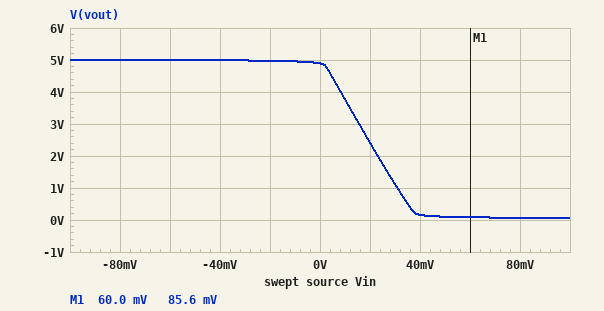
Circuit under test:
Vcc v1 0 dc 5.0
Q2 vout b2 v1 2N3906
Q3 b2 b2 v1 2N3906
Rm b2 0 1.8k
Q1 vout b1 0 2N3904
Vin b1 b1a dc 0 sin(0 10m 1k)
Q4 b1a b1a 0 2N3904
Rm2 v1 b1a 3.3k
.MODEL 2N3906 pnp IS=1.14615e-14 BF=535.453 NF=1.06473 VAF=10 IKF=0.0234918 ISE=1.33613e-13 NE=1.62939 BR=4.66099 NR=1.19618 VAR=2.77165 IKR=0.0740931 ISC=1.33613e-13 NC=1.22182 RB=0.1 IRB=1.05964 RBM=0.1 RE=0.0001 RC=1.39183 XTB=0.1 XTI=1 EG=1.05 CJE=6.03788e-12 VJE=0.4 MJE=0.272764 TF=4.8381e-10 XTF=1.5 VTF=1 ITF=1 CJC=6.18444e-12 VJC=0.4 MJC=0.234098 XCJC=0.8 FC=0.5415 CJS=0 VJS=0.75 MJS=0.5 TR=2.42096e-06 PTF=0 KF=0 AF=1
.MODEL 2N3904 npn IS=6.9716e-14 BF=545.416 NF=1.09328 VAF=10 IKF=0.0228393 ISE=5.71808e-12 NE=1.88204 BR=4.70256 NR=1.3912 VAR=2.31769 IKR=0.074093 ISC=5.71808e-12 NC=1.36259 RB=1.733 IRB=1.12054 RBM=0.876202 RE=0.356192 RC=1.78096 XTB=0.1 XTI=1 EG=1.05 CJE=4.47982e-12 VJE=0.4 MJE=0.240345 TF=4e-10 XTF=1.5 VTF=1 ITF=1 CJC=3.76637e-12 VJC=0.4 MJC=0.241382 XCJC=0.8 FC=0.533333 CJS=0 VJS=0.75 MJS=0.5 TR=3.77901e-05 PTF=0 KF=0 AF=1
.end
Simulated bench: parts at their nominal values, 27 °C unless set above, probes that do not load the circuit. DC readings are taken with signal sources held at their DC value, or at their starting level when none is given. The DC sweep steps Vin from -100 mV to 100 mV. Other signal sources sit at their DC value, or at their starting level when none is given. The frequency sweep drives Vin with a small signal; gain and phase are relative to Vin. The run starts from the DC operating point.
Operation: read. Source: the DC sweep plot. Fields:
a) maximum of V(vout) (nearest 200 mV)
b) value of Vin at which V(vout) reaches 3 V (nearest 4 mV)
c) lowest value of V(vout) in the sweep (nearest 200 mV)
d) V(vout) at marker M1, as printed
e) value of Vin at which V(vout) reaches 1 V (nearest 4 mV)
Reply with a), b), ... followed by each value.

a) 5.0 V
b) 16 mV
c) 0 V
d) 85.6 mV
e) 32 mV
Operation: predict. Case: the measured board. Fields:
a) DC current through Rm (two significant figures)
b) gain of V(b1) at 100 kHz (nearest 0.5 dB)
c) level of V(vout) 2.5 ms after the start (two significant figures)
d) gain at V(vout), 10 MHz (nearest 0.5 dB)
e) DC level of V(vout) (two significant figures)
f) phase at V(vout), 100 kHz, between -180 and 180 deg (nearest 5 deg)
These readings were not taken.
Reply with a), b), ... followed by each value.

a) 2.4 mA
b) 0 dB
c) 4.9 V
d) 1.0 dB
e) 4.9 V
f) 170 deg
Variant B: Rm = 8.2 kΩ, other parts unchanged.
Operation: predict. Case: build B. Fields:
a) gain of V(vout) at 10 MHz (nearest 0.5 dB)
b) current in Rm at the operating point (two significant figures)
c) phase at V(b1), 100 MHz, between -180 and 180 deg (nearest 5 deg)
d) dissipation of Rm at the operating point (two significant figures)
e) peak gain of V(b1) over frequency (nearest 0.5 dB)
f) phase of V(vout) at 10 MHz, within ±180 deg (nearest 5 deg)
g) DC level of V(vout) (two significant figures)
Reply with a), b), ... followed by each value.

a) -5.5 dB
b) 530 µA
c) 0 deg
d) 2.3 mW
e) -5.0 dB
f) 15 deg
g) 68 mV
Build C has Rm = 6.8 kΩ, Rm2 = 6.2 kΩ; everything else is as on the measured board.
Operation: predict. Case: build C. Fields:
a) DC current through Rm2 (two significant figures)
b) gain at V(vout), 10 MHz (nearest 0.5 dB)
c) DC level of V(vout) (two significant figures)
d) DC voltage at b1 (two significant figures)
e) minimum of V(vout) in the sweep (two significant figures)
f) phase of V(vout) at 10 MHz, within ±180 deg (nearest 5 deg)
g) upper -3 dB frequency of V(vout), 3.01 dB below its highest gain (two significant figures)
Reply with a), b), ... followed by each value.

a) 700 µA
b) 29.0 dB
c) 2.0 V
d) 660 mV
e) 40 mV
f) 100 deg
g) 1.9 MHz
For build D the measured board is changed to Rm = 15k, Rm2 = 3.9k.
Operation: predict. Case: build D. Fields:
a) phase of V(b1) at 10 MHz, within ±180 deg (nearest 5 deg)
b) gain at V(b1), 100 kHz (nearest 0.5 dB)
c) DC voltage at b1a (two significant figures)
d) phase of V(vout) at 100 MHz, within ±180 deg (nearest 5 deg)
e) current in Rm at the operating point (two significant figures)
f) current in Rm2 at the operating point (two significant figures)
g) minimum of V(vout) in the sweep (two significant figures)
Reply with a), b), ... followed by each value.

a) 0 deg
b) -5.5 dB
c) 670 mV
d) -5 deg
e) 290 µA
f) 1.1 mA
g) 19 mV
